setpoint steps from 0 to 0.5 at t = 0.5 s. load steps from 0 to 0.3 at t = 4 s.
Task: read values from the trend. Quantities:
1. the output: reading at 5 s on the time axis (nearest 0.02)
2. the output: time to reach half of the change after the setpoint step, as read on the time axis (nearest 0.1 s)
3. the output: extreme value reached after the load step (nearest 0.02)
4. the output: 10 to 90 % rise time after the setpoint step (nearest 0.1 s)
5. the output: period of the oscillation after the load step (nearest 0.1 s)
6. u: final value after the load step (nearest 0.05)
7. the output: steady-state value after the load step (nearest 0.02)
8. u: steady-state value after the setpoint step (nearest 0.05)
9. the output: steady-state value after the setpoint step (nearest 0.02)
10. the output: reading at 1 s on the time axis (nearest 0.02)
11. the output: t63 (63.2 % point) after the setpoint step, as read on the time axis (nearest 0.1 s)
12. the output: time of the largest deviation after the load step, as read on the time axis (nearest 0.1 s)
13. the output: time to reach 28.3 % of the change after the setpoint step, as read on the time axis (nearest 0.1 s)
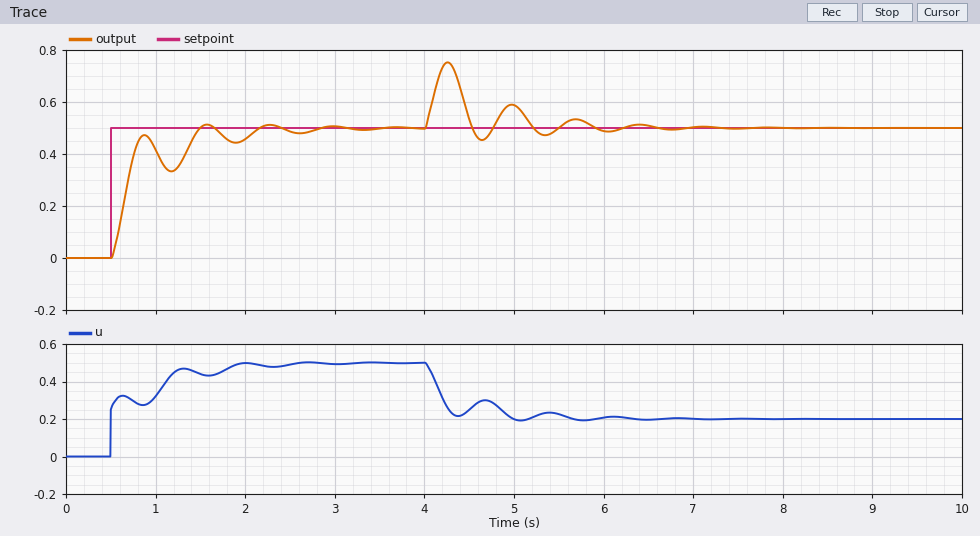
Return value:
0.58
0.7 s
0.76
0.3 s
0.7 s
0.20
0.50
0.50
0.50
0.42
0.7 s
4.3 s
0.6 s
